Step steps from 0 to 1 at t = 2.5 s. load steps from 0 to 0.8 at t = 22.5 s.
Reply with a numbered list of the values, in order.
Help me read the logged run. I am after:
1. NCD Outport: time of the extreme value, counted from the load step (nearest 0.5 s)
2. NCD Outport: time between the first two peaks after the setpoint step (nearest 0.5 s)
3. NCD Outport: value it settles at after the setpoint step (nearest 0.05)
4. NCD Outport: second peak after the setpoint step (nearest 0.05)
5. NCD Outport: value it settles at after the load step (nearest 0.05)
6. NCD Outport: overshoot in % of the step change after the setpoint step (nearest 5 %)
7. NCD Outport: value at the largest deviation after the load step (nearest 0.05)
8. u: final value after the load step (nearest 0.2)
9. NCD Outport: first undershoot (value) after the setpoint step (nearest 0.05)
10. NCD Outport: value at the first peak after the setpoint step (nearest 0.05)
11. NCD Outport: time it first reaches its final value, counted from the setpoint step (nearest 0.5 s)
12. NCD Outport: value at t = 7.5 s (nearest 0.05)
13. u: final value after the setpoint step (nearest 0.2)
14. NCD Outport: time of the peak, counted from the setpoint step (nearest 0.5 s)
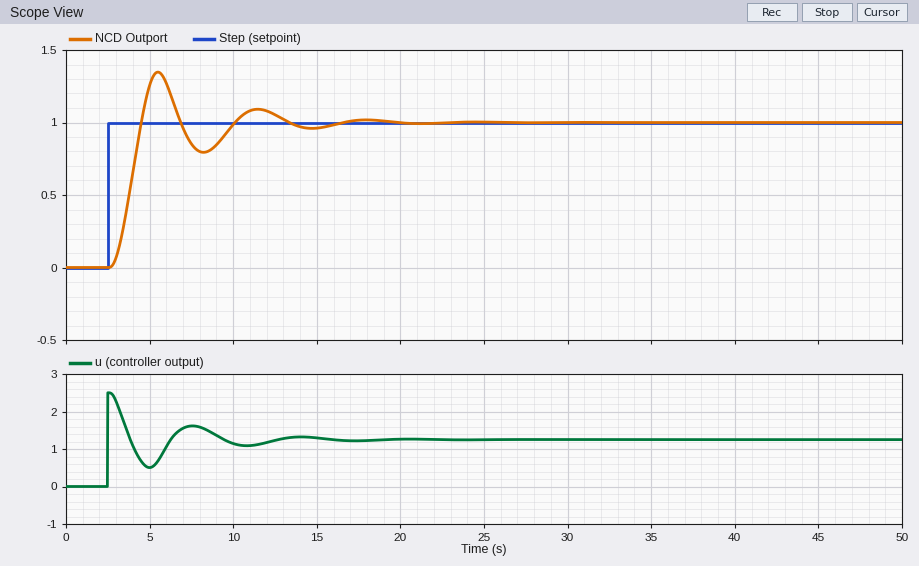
1. 2.0 s
2. 6.0 s
3. 1.00
4. 1.10
5. 1.00
6. 35 %
7. 1.00
8. 1.2
9. 0.80
10. 1.35
11. 2.0 s
12. 0.85
13. 1.2
14. 3.0 s
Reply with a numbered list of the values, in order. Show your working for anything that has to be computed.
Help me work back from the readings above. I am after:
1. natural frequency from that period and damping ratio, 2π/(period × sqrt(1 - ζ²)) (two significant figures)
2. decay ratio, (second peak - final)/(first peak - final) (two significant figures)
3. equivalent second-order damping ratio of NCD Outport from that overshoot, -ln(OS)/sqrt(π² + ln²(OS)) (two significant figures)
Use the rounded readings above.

1. 2π / (6 × sqrt(1 - 0.32²)) = 1.1 rad/s
2. (1.1 - 1) / (1.35 - 1) = 0.29
3. ln(0.35) = -1.050; 1.050 / sqrt(9.870 + 1.102) = 0.32
